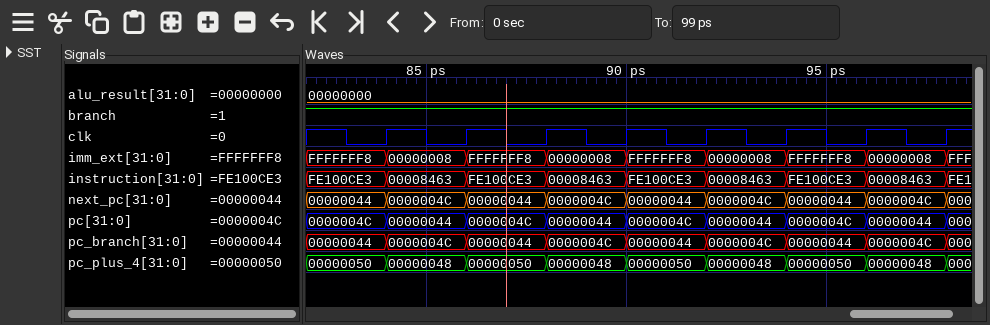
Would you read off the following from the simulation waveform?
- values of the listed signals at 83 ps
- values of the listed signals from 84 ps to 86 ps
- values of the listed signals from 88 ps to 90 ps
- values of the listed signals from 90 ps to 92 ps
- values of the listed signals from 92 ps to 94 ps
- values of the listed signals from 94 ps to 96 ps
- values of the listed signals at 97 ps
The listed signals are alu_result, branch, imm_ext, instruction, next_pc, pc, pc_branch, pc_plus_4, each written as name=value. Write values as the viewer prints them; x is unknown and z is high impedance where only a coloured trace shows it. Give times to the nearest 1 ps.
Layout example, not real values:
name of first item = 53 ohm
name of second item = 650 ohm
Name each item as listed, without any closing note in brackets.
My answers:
values of the listed signals at 83 ps = alu_result=00000000, branch=1, imm_ext=FFFFFFF8, instruction=FE100CE3, next_pc=00000044, pc=0000004C, pc_branch=00000044, pc_plus_4=00000050
values of the listed signals from 84 ps to 86 ps = alu_result=00000000, branch=1, imm_ext=00000008, instruction=00008463, next_pc=0000004C, pc=00000044, pc_branch=0000004C, pc_plus_4=00000048
values of the listed signals from 88 ps to 90 ps = alu_result=00000000, branch=1, imm_ext=00000008, instruction=00008463, next_pc=0000004C, pc=00000044, pc_branch=0000004C, pc_plus_4=00000048
values of the listed signals from 90 ps to 92 ps = alu_result=00000000, branch=1, imm_ext=FFFFFFF8, instruction=FE100CE3, next_pc=00000044, pc=0000004C, pc_branch=00000044, pc_plus_4=00000050
values of the listed signals from 92 ps to 94 ps = alu_result=00000000, branch=1, imm_ext=00000008, instruction=00008463, next_pc=0000004C, pc=00000044, pc_branch=0000004C, pc_plus_4=00000048
values of the listed signals from 94 ps to 96 ps = alu_result=00000000, branch=1, imm_ext=FFFFFFF8, instruction=FE100CE3, next_pc=00000044, pc=0000004C, pc_branch=00000044, pc_plus_4=00000050
values of the listed signals at 97 ps = alu_result=00000000, branch=1, imm_ext=00000008, instruction=00008463, next_pc=0000004C, pc=00000044, pc_branch=0000004C, pc_plus_4=00000048
